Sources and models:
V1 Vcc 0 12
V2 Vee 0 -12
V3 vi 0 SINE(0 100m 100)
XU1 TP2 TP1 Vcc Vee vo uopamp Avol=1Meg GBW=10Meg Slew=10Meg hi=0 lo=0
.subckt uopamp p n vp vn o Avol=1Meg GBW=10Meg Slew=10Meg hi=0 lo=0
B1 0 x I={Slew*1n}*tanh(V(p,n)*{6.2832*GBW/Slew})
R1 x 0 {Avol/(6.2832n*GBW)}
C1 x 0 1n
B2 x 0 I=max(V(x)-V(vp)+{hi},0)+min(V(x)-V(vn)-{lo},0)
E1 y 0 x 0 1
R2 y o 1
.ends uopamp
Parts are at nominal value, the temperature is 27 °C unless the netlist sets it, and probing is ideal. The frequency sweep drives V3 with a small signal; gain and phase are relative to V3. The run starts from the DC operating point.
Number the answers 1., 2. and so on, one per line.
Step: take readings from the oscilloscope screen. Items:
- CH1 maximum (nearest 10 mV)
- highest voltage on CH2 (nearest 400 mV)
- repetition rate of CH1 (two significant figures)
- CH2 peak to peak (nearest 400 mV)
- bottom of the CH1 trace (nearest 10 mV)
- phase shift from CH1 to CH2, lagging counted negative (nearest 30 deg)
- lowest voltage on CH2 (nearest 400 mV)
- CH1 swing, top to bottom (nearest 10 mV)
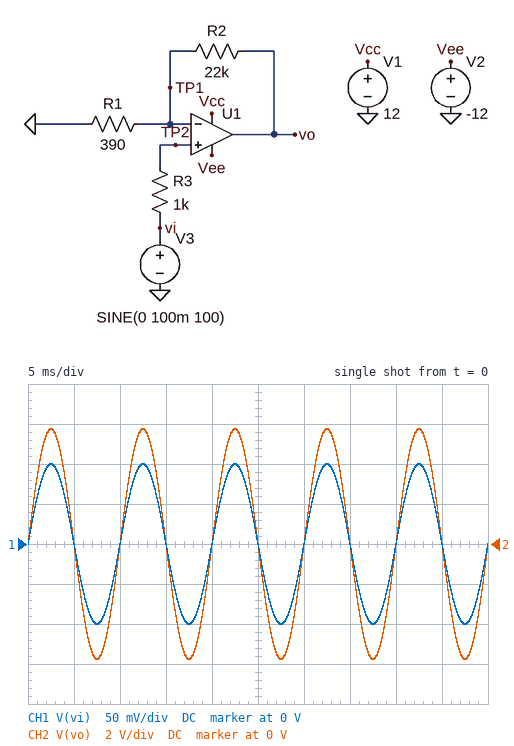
1. 100 mV
2. 5.6 V
3. 100 Hz
4. 11.6 V
5. -100 mV
6. 0 deg
7. -5.6 V
8. 200 mV
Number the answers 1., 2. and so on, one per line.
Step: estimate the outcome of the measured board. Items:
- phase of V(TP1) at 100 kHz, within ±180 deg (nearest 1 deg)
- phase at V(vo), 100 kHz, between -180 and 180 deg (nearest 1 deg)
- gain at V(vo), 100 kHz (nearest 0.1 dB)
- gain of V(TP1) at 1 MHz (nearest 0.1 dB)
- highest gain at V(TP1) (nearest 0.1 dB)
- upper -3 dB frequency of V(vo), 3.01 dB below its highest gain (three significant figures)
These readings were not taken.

1. -30 deg
2. -30 deg
3. 33.9 dB
4. -15.3 dB
5. 0 dB
6. 174 kHz
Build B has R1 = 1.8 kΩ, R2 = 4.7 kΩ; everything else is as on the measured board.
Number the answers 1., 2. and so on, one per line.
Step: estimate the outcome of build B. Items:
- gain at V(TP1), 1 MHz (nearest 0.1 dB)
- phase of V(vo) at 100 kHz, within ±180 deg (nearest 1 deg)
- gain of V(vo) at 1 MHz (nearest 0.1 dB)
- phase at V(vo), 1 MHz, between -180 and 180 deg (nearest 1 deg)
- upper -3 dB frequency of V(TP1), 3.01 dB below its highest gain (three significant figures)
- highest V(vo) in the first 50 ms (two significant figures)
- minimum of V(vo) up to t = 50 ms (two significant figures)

1. -0.5 dB
2. -2 deg
3. 10.6 dB
4. -20 deg
5. 2.77 MHz
6. 360 mV
7. -360 mV
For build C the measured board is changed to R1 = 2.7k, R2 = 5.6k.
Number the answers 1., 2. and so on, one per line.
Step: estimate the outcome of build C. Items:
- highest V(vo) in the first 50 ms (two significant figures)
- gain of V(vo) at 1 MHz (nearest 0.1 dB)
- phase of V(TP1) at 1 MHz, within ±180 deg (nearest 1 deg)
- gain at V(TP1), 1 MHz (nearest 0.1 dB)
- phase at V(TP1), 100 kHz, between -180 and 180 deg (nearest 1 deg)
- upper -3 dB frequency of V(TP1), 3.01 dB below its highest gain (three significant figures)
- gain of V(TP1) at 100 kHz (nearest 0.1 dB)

1. 310 mV
2. 9.4 dB
3. -17 deg
4. -0.4 dB
5. -2 deg
6. 3.25 MHz
7. 0 dB
